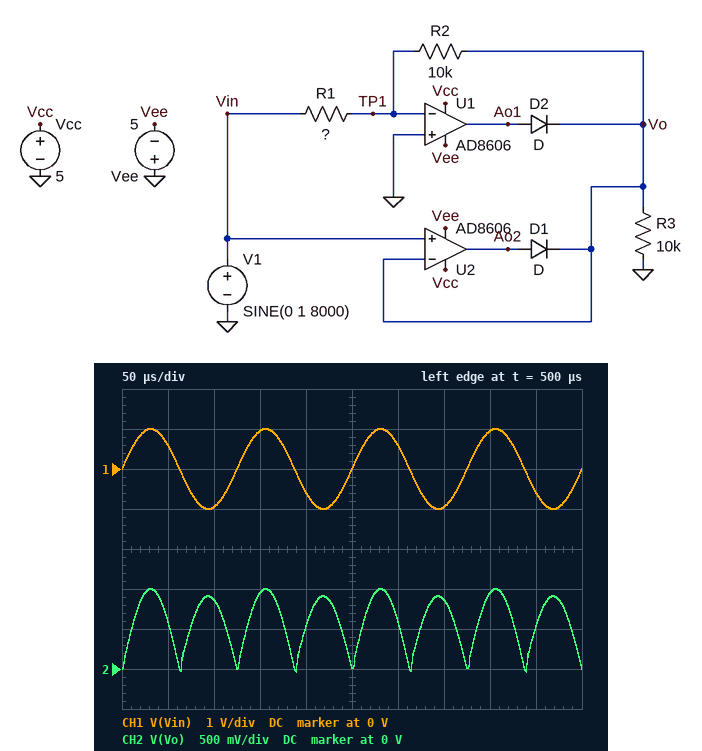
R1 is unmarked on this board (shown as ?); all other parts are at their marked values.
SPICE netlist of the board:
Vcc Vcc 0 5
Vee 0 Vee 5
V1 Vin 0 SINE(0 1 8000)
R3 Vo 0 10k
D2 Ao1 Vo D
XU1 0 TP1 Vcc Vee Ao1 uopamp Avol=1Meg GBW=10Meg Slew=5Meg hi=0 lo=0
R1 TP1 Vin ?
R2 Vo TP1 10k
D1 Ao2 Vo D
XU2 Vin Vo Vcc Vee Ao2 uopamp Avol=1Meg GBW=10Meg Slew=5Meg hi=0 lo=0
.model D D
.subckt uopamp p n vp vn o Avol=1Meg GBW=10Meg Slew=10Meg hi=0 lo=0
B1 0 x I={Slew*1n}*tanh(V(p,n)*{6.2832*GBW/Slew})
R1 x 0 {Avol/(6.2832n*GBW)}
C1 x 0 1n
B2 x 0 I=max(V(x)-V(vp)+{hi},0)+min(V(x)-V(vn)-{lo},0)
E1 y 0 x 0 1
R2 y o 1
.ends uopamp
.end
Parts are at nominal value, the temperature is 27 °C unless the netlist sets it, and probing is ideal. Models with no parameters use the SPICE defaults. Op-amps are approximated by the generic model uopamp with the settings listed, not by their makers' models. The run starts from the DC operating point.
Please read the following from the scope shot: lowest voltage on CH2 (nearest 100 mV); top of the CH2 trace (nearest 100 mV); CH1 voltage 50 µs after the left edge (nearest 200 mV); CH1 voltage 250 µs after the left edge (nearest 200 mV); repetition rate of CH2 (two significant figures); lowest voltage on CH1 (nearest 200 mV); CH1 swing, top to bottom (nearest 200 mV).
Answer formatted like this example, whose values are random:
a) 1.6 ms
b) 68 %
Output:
a) 0 V
b) 1.0 V
c) 600 mV
d) 0 V
e) 16 kHz
f) -1.0 V
g) 2.0 V
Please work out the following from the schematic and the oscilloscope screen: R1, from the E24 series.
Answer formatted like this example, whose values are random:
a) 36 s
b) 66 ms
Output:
a) 11 kΩ
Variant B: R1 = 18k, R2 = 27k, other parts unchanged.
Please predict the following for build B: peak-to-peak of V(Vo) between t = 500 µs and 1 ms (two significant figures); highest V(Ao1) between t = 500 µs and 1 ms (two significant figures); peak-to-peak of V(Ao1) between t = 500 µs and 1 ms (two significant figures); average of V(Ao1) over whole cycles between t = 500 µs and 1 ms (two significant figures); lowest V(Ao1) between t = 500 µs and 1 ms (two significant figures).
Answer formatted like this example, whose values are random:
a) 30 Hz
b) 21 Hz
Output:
a) 1.5 V
b) 2.1 V
c) 7.1 V
d) -1.7 V
e) -5.0 V
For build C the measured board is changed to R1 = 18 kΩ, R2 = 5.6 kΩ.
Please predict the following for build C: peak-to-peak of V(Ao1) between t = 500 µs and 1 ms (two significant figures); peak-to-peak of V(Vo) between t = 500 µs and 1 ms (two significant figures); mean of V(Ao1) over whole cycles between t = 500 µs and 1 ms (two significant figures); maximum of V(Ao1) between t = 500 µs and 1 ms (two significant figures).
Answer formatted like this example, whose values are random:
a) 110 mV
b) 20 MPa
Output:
a) 5.9 V
b) 1.0 V
c) -2.1 V
d) 900 mV
